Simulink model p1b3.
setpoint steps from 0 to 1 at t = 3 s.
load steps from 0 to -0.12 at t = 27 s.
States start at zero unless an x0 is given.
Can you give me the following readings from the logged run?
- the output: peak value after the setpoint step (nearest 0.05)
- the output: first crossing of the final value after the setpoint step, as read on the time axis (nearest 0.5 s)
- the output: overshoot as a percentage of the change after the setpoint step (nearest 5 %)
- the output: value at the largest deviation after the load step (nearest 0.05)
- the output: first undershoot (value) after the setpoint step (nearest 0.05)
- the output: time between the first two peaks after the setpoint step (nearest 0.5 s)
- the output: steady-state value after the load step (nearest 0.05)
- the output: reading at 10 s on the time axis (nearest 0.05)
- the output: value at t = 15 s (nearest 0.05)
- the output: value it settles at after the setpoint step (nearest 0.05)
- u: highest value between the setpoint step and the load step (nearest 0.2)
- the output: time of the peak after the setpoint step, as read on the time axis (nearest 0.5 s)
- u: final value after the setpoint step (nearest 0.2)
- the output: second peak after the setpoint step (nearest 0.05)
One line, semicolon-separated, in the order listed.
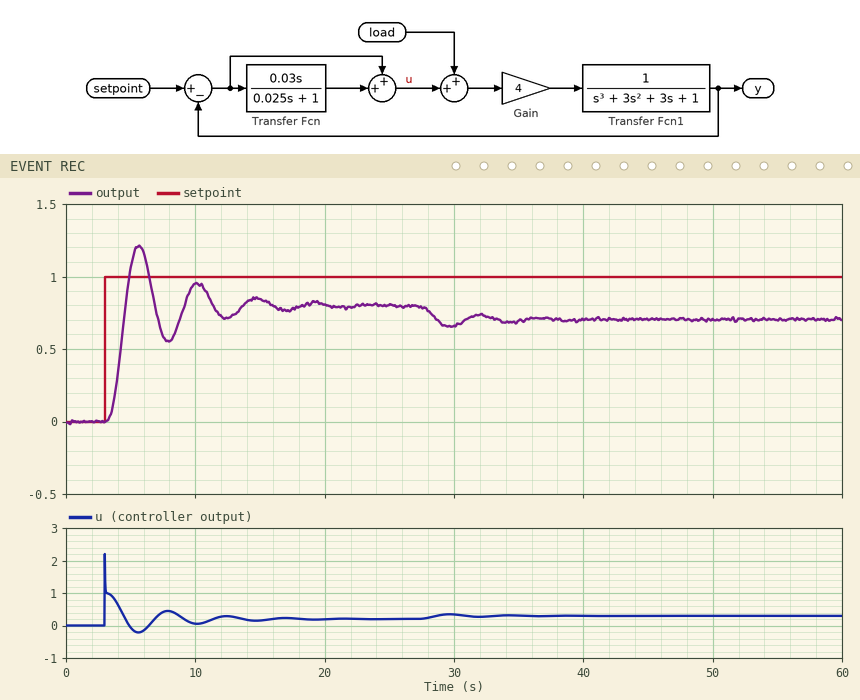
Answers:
1.20; 4.5 s; 50 %; 0.65; 0.55; 4.5 s; 0.70; 0.95; 0.85; 0.80; 2.2; 5.5 s; 0.2; 0.95
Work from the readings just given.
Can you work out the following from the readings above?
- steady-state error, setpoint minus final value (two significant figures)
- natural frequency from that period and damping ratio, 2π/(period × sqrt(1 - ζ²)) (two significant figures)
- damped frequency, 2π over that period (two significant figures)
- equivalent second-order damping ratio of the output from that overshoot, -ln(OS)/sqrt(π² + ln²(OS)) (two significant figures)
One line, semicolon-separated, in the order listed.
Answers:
0.20; 1.4 rad/s; 1.4 rad/s; 0.22
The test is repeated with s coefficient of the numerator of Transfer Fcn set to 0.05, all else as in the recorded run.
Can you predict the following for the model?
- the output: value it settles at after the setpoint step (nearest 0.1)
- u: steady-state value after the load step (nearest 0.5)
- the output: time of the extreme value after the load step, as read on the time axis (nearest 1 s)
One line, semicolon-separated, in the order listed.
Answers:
0.8; 0.5; 30 s
